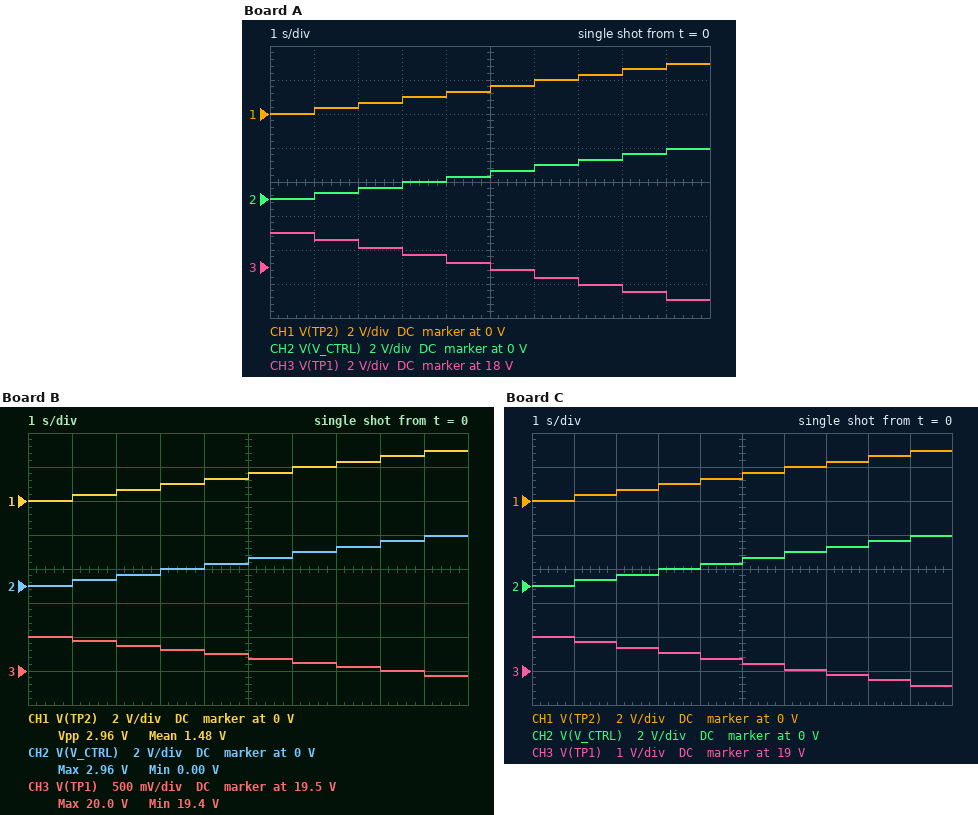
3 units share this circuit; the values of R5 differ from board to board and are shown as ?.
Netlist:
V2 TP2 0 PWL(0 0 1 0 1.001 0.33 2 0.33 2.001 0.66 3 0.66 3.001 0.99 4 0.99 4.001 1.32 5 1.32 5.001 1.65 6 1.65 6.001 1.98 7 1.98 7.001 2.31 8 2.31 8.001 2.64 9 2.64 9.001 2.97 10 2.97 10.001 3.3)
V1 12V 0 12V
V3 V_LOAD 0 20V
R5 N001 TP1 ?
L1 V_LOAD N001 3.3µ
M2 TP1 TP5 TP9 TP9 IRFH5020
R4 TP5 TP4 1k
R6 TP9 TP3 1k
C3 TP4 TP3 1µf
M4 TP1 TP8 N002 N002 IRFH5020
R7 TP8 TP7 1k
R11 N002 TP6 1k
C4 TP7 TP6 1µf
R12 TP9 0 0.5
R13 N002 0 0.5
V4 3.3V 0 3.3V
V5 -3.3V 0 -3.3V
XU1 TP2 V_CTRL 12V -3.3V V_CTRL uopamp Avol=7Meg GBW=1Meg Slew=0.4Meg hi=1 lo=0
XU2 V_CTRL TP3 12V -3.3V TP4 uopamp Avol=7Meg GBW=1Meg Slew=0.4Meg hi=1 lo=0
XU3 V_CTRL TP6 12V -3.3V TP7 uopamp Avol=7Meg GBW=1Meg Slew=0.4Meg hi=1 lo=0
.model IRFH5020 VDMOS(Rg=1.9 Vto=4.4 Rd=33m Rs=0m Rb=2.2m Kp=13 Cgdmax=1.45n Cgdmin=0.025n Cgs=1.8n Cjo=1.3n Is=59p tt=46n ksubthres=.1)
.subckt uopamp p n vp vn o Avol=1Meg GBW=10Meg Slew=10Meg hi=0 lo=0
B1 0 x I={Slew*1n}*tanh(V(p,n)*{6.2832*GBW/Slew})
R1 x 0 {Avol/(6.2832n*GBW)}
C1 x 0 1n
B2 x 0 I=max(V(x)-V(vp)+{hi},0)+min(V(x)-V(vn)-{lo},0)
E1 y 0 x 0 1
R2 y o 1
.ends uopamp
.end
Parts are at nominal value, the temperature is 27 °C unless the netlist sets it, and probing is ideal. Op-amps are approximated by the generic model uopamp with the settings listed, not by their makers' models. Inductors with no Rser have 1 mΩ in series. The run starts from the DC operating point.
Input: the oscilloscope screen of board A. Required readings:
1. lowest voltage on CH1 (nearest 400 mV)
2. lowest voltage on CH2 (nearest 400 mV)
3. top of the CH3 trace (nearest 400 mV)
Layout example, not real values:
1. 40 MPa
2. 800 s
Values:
1. 0 V
2. 0 V
3. 20.0 V
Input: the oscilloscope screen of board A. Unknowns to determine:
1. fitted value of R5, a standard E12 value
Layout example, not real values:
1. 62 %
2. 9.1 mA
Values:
1. 0.33 Ω
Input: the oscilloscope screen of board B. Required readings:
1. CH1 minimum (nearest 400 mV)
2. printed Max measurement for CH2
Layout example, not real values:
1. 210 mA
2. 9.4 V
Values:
1. 0 V
2. 2.96 V
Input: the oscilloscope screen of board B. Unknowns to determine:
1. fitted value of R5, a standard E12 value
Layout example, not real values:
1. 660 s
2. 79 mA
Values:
1. 0.047 Ω
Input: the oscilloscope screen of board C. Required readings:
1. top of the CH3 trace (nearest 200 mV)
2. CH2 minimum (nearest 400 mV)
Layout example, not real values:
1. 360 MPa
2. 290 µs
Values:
1. 20.0 V
2. 0 V
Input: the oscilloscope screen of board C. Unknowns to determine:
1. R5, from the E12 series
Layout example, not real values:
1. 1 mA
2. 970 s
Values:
1. 0.12 Ω
